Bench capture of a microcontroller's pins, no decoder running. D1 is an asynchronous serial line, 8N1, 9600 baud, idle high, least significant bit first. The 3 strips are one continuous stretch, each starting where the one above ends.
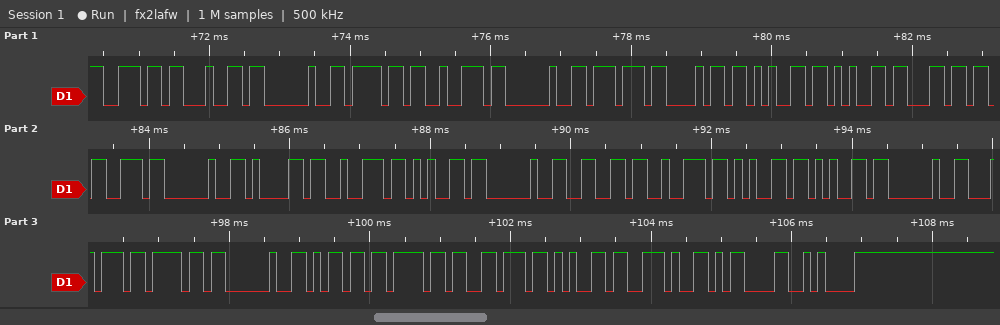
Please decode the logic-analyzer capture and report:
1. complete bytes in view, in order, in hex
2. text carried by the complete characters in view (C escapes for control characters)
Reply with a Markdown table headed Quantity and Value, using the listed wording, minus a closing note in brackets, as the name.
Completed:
| Quantity | Value |
|---|---|
| complete bytes in view, in order, in hex | 0x6E 0x64 0x20 0x6F 0x72 0x20 0x77 0x68 0x65 0x65 0x6C 0x73 0x20 0x61 0x72 0x65 0x20 0x66 0x72 0x65 0x65 0x20 0x74 0x6F 0x20 0x6D 0x6F 0x76 0x65 0x2E 0x0D 0x0A |
| text carried by the complete characters in view | "nd or wheels are free to move.\r\n" |
